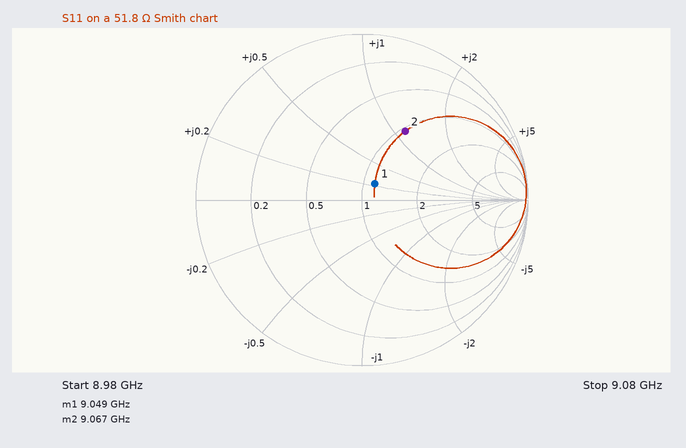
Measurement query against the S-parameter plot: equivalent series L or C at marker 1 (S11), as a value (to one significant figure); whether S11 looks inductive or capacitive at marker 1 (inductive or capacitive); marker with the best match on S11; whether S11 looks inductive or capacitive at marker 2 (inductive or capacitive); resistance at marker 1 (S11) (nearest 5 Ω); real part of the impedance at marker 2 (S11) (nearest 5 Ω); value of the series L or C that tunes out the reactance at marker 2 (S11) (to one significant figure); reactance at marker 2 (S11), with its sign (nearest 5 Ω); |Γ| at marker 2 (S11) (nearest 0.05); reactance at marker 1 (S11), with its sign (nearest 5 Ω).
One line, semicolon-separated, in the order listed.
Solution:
200 pH; inductive; marker 1; inductive; 60 Ω; 55 Ω; 300 fF; +60 Ω; 0.50; +10 Ω
